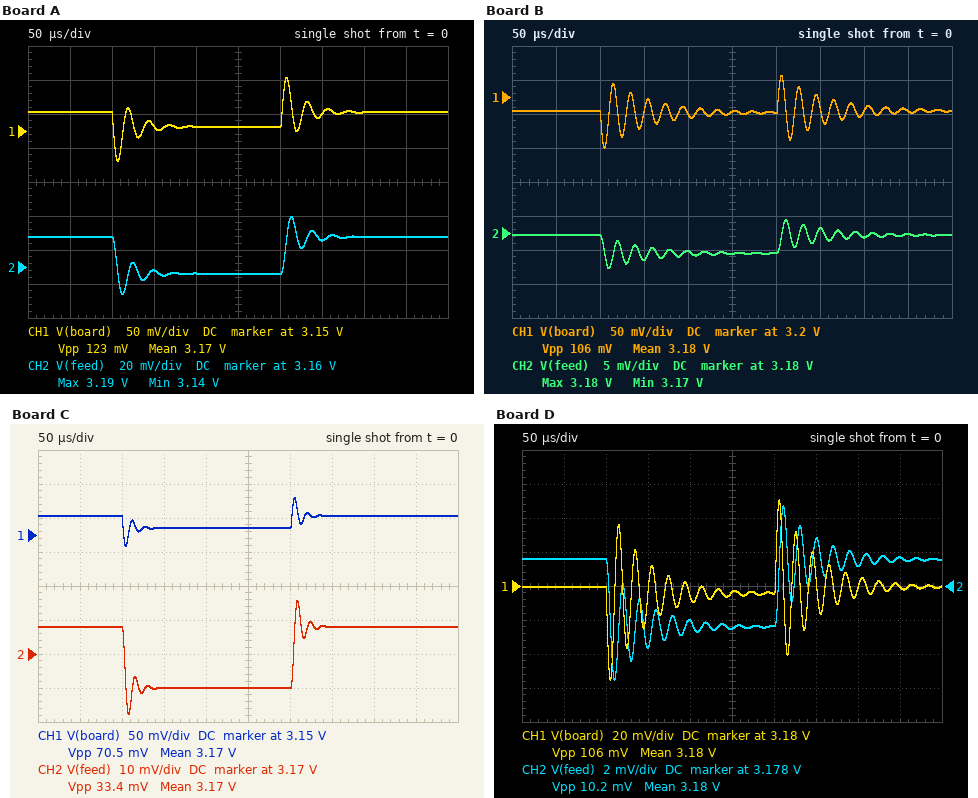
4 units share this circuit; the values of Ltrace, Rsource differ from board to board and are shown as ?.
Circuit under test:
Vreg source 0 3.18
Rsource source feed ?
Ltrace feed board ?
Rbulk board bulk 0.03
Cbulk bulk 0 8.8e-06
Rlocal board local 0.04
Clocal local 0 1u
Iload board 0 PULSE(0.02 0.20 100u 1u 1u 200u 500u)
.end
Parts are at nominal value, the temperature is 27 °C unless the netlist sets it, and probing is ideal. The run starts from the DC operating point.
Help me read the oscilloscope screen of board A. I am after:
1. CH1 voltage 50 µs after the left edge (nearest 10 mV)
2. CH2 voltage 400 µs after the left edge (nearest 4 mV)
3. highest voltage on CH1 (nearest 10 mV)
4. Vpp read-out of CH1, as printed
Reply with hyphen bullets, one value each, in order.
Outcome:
- 3.18 V
- 3.176 V
- 3.23 V
- 123 mV
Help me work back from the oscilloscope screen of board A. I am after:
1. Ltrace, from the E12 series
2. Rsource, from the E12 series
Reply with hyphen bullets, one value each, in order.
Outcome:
- 1.5 µH
- 0.12 Ω
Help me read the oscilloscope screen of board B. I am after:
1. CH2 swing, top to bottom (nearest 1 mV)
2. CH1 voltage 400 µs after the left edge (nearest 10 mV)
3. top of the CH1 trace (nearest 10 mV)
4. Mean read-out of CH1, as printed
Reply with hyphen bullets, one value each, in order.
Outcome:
- 7 mV
- 3.18 V
- 3.23 V
- 3.18 V
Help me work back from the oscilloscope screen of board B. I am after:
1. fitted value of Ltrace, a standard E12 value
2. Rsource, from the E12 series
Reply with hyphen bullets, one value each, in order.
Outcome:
- 1 µH
- 0.015 Ω
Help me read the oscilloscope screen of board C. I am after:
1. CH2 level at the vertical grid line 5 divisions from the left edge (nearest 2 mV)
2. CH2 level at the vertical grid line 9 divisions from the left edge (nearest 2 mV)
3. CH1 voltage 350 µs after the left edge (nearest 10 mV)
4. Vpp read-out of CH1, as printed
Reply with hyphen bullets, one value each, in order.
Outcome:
- 3.160 V
- 3.178 V
- 3.18 V
- 70.5 mV
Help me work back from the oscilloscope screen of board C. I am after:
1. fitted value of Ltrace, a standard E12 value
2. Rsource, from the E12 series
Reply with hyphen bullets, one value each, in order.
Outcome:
- 560 nH
- 0.1 Ω
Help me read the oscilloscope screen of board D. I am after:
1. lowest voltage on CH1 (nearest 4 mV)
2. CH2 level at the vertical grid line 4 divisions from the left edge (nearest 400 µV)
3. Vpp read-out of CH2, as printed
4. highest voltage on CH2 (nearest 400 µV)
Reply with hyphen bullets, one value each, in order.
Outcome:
- 3.124 V
- 3.1760 V
- 10.2 mV
- 3.1828 V
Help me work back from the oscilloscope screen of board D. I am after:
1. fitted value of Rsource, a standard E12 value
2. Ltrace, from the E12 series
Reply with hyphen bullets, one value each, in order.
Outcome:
- 0.022 Ω
- 1 µH
